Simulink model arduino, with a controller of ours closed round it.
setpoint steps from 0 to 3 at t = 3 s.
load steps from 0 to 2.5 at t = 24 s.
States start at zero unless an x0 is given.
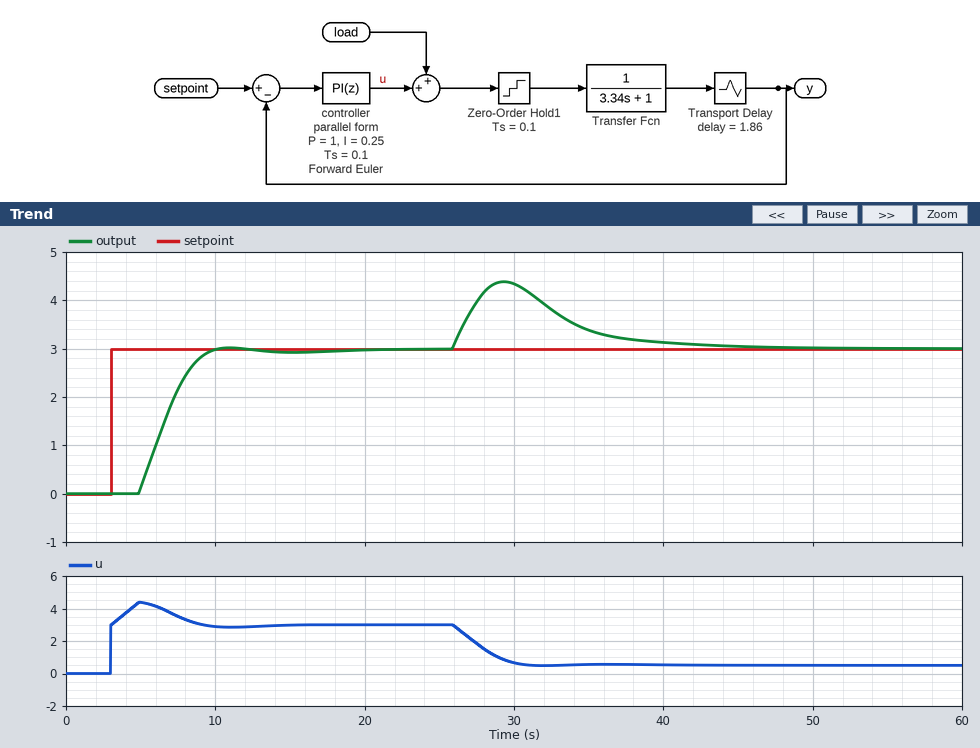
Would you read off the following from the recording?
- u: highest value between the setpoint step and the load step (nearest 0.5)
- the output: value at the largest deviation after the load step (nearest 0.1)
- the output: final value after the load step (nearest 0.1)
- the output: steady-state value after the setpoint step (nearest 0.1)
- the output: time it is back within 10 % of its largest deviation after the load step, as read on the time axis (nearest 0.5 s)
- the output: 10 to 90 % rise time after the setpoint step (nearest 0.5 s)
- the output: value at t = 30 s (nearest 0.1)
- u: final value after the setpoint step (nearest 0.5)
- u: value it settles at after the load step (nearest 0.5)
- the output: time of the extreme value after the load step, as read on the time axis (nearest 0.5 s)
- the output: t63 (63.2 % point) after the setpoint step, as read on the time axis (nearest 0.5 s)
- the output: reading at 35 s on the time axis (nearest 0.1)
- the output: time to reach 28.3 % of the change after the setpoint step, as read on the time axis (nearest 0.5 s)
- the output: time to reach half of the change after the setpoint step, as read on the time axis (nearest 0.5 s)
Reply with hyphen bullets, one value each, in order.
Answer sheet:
- 4.5
- 4.4
- 3.0
- 3.0
- 39.5 s
- 3.5 s
- 4.3
- 3.0
- 0.5
- 29.5 s
- 7.0 s
- 3.4
- 6.0 s
- 6.5 s
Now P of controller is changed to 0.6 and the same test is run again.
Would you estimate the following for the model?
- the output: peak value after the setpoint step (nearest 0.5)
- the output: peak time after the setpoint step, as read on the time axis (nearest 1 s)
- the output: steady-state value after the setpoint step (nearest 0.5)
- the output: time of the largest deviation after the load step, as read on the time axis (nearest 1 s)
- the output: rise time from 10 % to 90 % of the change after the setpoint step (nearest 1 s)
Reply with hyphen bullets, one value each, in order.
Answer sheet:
- 3.5
- 15 s
- 3.0
- 30 s
- 5 s
